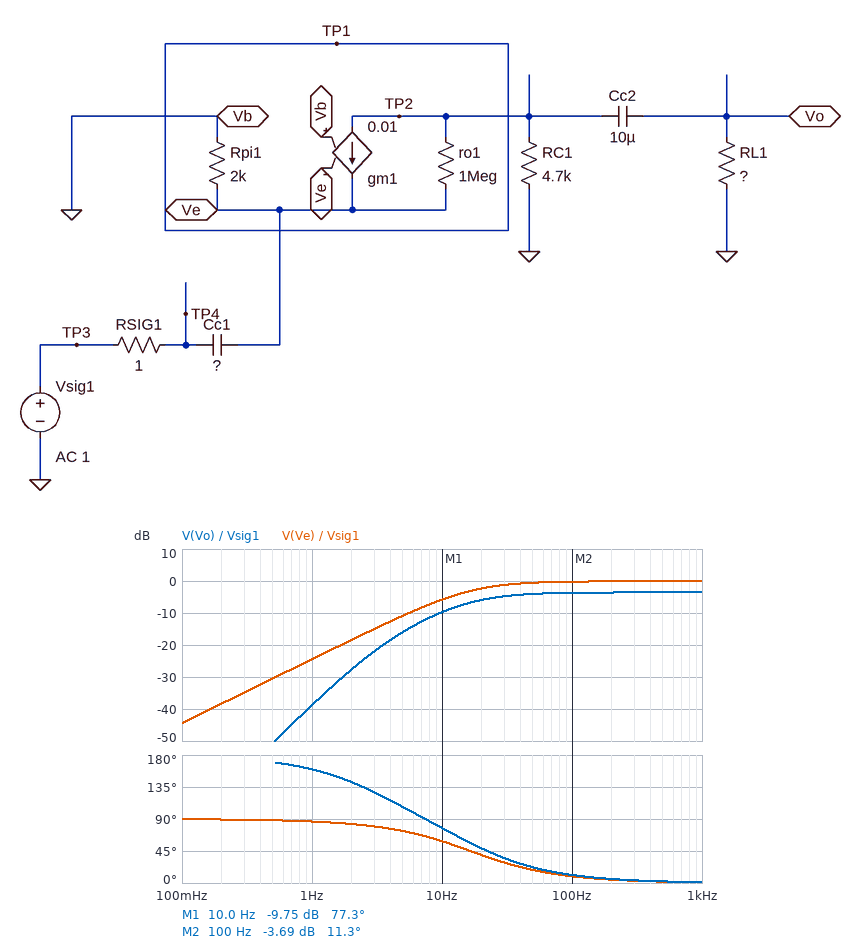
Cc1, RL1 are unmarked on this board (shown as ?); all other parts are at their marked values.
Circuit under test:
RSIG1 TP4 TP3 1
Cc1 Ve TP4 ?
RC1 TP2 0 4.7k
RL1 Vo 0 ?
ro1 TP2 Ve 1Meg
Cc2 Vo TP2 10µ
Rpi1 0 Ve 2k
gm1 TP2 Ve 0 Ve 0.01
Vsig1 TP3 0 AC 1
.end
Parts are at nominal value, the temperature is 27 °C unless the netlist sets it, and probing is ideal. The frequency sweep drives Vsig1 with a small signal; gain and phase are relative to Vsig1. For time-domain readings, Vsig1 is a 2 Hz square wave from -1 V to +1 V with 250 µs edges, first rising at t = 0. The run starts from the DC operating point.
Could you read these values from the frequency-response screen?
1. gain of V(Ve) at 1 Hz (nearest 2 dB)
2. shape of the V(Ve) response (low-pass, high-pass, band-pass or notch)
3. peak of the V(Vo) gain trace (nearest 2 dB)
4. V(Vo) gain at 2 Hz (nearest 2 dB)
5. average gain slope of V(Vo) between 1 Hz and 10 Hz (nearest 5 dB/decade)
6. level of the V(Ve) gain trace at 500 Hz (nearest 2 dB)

-24 dB
high-pass
-4 dB
-28 dB
30 dB/decade
0 dB
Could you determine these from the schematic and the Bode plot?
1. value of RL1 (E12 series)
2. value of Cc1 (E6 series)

68 Ω
100 µF
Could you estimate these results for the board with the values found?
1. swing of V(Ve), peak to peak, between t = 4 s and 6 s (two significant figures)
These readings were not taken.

3.9 V
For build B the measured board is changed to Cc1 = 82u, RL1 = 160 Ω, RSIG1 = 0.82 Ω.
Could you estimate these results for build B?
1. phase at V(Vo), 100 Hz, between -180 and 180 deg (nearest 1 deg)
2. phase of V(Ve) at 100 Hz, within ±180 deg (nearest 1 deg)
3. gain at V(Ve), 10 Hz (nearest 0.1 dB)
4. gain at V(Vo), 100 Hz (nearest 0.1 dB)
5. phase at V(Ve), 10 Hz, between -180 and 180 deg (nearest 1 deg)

13 deg
11 deg
-7.1 dB
3.5 dB
64 deg
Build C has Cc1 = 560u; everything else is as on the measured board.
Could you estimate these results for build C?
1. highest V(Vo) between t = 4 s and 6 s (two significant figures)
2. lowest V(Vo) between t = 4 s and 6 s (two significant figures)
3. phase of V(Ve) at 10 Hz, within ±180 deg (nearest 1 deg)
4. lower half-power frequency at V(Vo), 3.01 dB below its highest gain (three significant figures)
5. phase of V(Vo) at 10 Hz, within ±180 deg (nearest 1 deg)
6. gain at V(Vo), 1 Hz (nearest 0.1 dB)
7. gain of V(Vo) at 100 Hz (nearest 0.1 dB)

1.4 V
-1.4 V
16 deg
4.91 Hz
35 deg
-24.3 dB
-3.6 dB
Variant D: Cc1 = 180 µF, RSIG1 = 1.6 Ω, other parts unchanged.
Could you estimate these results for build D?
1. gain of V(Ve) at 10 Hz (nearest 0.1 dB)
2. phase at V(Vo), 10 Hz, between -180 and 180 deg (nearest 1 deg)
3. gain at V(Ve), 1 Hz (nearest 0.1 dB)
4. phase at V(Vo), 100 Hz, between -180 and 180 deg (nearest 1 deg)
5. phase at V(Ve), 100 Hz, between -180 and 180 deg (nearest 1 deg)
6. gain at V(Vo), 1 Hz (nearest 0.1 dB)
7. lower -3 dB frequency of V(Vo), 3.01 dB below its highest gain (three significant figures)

-2.8 dB
61 deg
-19.4 dB
7 deg
5 deg
-33.7 dB
10.2 Hz
